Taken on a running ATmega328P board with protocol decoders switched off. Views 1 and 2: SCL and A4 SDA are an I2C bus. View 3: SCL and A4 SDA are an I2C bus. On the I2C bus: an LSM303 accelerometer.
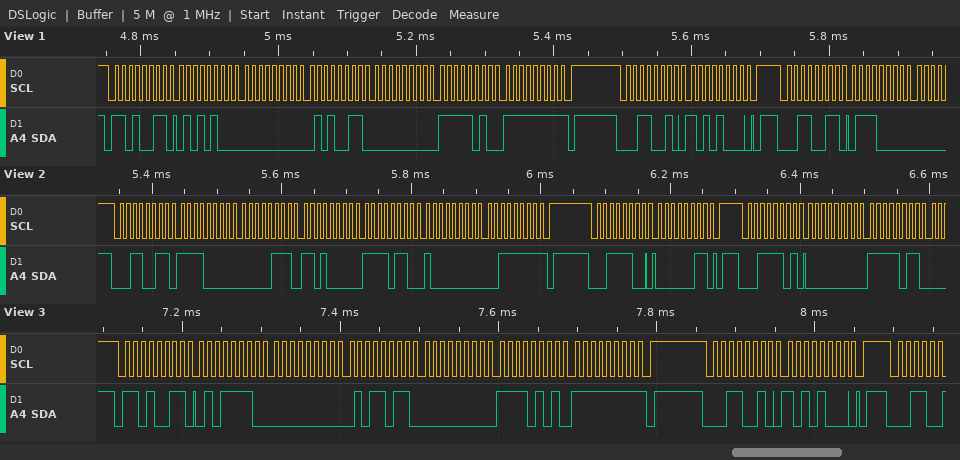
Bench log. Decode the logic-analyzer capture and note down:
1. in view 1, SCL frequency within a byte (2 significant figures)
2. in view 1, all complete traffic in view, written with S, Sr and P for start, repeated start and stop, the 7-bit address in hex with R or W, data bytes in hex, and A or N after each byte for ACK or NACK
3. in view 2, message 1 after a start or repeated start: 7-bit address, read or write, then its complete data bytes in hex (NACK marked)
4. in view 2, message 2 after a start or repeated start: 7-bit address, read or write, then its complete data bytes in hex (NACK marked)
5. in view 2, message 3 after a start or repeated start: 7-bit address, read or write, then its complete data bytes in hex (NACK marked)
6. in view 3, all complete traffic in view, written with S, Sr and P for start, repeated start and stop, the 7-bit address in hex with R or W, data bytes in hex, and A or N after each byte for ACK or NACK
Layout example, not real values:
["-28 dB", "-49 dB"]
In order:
["100 kHz", "S 69R A 54 A 00 A 53 A 00 A FA A FF N P S 19W A A8 A P S 19R A 70 A", "0x19 read: F0 07 D0 F6 80 3F NACK", "0x1E write: 03", "0x1E read: 00 FB", "S 69R A 5E A 00 A 5B A 00 A F5 A FF N P S 19W A A8 A P"]
